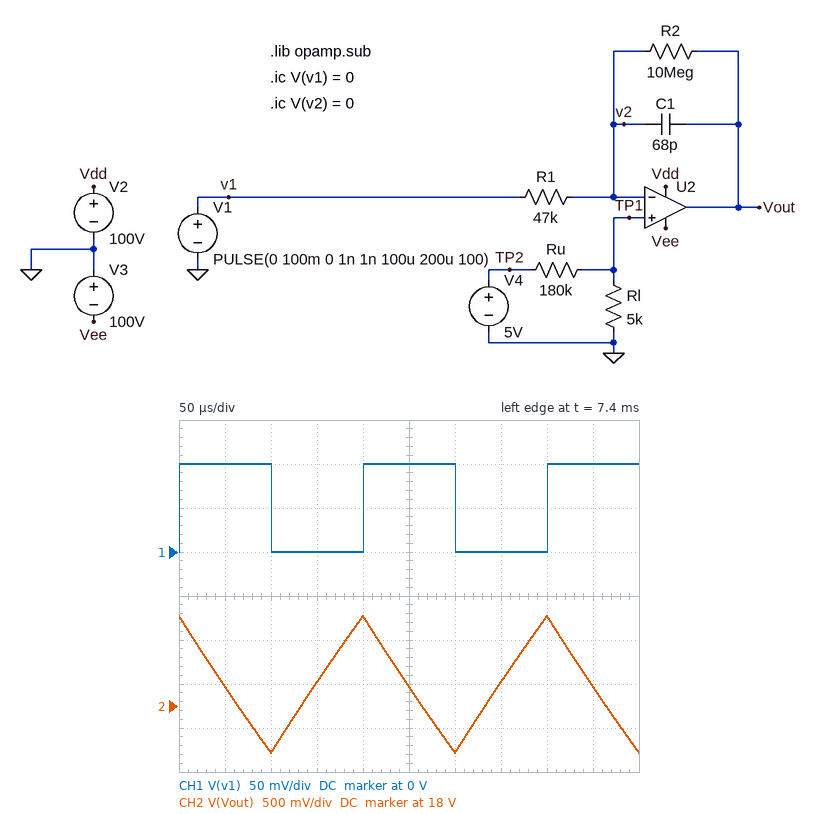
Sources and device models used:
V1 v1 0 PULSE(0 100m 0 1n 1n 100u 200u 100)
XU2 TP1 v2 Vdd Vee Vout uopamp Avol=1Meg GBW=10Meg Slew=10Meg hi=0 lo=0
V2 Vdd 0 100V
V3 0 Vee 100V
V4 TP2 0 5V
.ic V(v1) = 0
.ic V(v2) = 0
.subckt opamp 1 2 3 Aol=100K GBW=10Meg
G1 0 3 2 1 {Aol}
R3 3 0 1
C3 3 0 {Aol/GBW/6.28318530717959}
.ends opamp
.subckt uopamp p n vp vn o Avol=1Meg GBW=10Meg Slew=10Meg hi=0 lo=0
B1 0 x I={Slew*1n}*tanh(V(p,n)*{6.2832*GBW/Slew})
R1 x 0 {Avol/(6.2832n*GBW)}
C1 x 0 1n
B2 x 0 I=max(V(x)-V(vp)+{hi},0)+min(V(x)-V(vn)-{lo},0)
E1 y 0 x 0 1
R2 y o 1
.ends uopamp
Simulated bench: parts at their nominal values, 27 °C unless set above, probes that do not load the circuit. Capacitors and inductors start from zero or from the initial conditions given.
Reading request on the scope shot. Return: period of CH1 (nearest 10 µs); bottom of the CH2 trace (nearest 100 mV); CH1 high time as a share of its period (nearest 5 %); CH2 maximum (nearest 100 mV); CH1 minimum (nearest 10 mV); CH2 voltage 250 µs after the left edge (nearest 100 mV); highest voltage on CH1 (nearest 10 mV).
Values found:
200 µs
17.5 V
50 %
19.0 V
0 V
18.2 V
100 mV
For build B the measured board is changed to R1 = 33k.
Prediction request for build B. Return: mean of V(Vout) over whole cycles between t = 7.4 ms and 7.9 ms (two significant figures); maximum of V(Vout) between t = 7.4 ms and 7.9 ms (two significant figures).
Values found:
26 V
27 V
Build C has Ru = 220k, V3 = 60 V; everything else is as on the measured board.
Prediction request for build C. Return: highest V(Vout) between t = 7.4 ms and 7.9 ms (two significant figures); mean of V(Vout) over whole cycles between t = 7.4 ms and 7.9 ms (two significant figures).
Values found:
14 V
13 V
